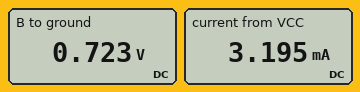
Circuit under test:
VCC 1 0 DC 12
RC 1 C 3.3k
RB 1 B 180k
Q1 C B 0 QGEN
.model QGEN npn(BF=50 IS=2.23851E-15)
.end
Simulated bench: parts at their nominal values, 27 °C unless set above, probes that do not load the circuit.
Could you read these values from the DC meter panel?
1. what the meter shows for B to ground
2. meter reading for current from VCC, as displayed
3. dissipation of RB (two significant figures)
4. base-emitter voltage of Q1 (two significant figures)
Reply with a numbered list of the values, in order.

1. 0.723 V
2. 3.195 mA
3. 710 µW
4. 720 mV
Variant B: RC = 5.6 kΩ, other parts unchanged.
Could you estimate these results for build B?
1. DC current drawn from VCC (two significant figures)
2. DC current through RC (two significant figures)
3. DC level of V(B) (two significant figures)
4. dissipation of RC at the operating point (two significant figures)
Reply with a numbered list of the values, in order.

1. 2.2 mA
2. 2.1 mA
3. 710 mV
4. 25 mW
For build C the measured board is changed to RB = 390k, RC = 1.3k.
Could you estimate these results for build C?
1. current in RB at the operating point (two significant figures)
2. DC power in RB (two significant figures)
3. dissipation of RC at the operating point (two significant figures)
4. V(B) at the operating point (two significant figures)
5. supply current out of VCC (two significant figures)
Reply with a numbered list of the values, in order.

1. 29 µA
2. 330 µW
3. 2.7 mW
4. 700 mV
5. 1.5 mA
